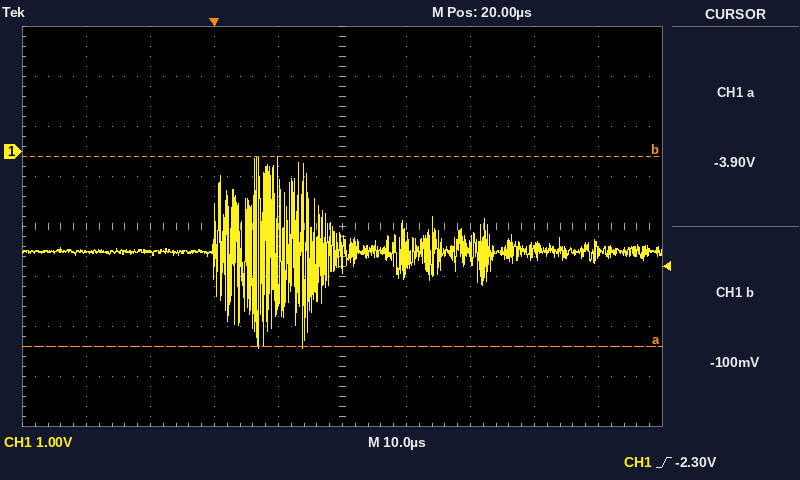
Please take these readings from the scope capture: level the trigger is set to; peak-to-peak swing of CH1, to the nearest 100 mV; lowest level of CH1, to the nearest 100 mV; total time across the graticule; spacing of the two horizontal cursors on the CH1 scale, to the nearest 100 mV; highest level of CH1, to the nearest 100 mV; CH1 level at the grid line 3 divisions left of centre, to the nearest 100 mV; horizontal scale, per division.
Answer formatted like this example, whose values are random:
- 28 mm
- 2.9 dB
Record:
- -2.30 V
- 3.8 V
- -3.9 V
- 100 µs
- 3.8 V
- -100 mV
- -2.0 V
- 10 µs
